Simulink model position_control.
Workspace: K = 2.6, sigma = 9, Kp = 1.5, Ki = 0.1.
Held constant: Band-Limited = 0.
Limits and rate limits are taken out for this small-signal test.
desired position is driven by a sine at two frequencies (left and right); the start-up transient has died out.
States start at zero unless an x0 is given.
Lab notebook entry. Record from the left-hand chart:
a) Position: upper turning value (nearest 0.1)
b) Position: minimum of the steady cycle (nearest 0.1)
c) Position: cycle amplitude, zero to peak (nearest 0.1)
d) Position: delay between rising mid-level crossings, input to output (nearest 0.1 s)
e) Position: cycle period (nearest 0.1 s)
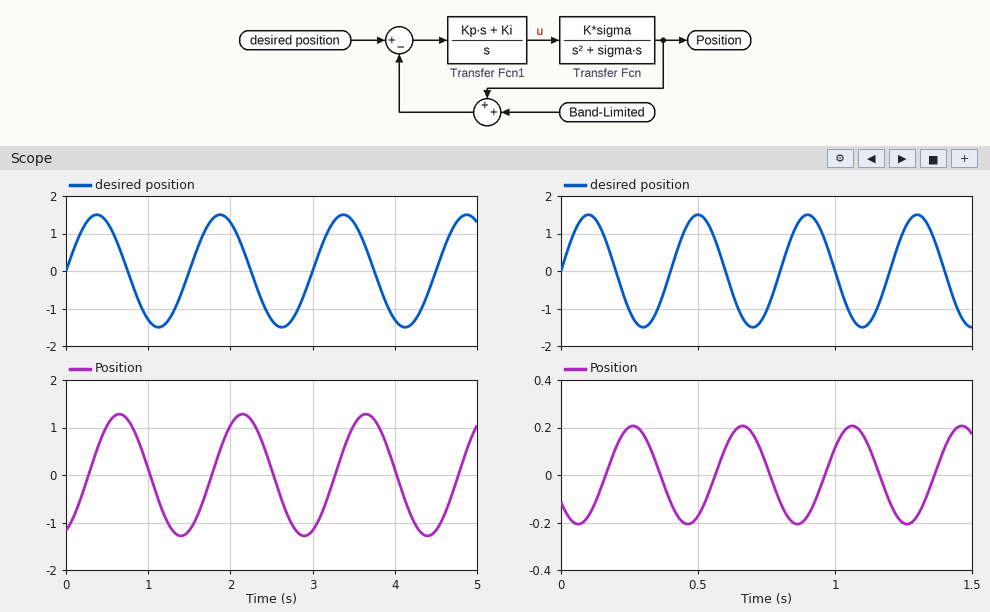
1.3
-1.3
1.3
0.3 s
1.5 s
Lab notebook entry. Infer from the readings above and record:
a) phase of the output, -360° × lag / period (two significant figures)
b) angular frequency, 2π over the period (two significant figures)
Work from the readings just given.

-72°
4.2 rad/s
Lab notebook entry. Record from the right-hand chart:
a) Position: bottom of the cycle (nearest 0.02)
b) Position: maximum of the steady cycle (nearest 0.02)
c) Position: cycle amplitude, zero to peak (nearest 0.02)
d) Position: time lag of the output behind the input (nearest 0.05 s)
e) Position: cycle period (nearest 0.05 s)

-0.20
0.20
0.20
0.15 s
0.40 s
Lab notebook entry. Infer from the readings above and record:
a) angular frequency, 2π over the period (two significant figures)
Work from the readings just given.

16 rad/s
